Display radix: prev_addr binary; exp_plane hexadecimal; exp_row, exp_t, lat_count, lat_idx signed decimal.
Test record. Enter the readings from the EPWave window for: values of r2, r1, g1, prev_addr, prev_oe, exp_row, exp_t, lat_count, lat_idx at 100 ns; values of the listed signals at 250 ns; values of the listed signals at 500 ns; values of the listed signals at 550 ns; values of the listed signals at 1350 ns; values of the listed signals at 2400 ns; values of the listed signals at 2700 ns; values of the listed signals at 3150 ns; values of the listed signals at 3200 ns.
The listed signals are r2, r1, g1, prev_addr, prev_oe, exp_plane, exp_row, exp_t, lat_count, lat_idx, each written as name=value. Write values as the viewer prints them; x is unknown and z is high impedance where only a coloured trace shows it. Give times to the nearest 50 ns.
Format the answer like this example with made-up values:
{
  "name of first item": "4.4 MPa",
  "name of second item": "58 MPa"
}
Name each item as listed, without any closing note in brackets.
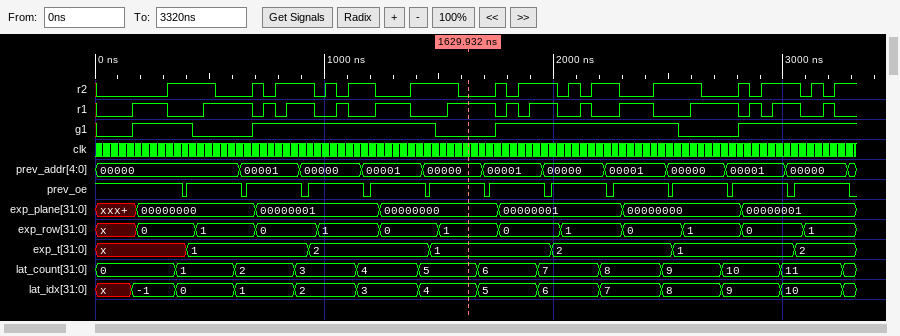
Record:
{
  "values of r2, r1, g1, prev_addr, prev_oe, exp_row, exp_t, lat_count, lat_idx at 100 ns": "r2=0, r1=0, g1=0, prev_addr=00000, prev_oe=1, exp_row=x, exp_t=x, lat_count=0, lat_idx=x",
  "values of the listed signals at 250 ns": "r2=0, r1=1, g1=1, prev_addr=00000, prev_oe=1, exp_plane=00000000, exp_row=0, exp_t=x, lat_count=0, lat_idx=-1",
  "values of the listed signals at 500 ns": "r2=1, r1=1, g1=0, prev_addr=00000, prev_oe=1, exp_plane=00000000, exp_row=1, exp_t=1, lat_count=1, lat_idx=0",
  "values of the listed signals at 550 ns": "r2=0, r1=1, g1=0, prev_addr=00000, prev_oe=1, exp_plane=00000000, exp_row=1, exp_t=1, lat_count=1, lat_idx=0",
  "values of the listed signals at 1350 ns": "r2=0, r1=1, g1=1, prev_addr=00001, prev_oe=1, exp_plane=00000000, exp_row=0, exp_t=2, lat_count=4, lat_idx=3",
  "values of the listed signals at 2400 ns": "r2=0, r1=1, g1=1, prev_addr=00001, prev_oe=1, exp_plane=00000000, exp_row=0, exp_t=2, lat_count=8, lat_idx=7",
  "values of the listed signals at 2700 ns": "r2=0, r1=1, g1=0, prev_addr=00000, prev_oe=1, exp_plane=00000000, exp_row=1, exp_t=1, lat_count=9, lat_idx=8",
  "values of the listed signals at 3150 ns": "r2=1, r1=0, g1=1, prev_addr=00000, prev_oe=1, exp_plane=00000001, exp_row=1, exp_t=2, lat_count=11, lat_idx=10",
  "values of the listed signals at 3200 ns": "r2=0, r1=1, g1=1, prev_addr=00000, prev_oe=1, exp_plane=00000001, exp_row=1, exp_t=2, lat_count=11, lat_idx=10"
}
